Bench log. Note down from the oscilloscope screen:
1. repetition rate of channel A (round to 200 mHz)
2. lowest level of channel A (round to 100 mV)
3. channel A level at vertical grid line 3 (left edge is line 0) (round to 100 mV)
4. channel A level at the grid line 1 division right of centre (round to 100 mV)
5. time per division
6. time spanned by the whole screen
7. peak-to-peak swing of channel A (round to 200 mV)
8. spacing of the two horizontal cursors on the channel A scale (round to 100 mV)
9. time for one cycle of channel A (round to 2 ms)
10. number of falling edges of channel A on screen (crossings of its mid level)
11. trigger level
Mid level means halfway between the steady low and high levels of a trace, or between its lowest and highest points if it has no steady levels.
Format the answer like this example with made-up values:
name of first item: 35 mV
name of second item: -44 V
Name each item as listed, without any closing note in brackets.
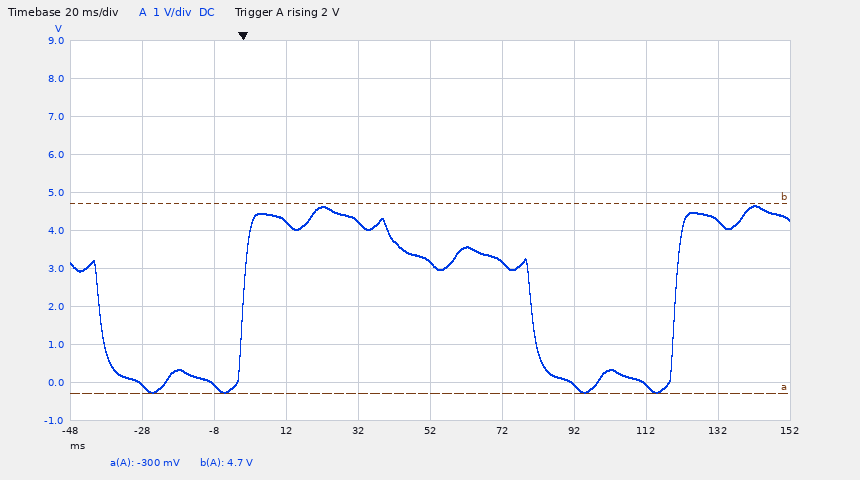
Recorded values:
repetition rate of channel A: 8.4 Hz
lowest level of channel A: -300 mV
channel A level at vertical grid line 3 (left edge is line 0): 4.2 V
channel A level at the grid line 1 division right of centre: 3.2 V
time per division: 20 ms
time spanned by the whole screen: 200 ms
peak-to-peak swing of channel A: 5.0 V
spacing of the two horizontal cursors on the channel A scale: 5.0 V
time for one cycle of channel A: 120 ms
number of falling edges of channel A on screen: 2
trigger level: 2 V
